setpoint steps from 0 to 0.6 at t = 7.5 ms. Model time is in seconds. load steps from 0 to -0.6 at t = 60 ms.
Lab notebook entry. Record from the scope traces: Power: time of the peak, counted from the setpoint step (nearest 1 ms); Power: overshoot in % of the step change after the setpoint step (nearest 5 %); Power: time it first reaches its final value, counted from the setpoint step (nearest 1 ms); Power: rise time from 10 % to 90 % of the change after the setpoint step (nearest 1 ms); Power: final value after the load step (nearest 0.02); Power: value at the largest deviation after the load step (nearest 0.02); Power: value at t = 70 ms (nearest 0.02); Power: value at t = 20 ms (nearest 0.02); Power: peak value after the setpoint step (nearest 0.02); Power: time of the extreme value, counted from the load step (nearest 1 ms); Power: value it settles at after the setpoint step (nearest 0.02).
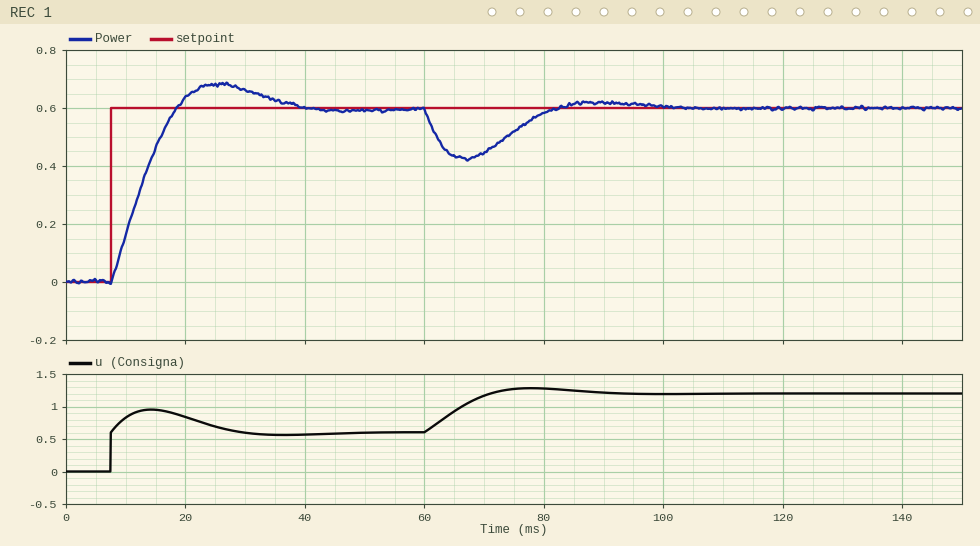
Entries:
18 ms
15 %
11 ms
8 ms
0.60
0.42
0.44
0.64
0.68
7 ms
0.60
